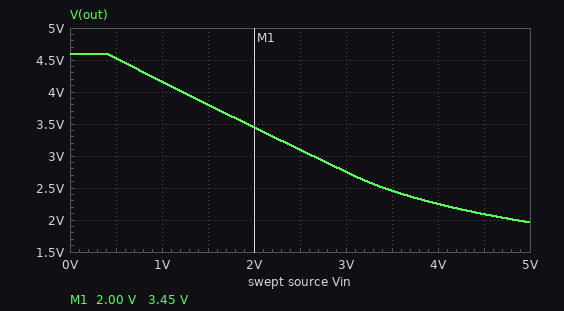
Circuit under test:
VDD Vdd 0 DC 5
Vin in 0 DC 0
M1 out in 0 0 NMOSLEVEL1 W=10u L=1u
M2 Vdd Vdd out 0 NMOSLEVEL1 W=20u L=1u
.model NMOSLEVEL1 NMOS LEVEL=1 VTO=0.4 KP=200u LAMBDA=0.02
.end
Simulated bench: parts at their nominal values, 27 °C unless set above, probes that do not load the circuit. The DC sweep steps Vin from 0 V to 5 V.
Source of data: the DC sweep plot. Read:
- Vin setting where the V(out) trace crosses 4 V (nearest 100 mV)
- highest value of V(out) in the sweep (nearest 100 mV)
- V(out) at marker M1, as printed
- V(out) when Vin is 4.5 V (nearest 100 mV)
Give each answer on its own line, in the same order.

1.2 V
4.6 V
3.45 V
2.1 V
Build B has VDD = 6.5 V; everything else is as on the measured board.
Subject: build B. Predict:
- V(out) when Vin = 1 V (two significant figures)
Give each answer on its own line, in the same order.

5.7 V
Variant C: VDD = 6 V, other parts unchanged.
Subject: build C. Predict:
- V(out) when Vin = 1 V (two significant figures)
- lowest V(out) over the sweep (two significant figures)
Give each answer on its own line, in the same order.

5.2 V
2.7 V
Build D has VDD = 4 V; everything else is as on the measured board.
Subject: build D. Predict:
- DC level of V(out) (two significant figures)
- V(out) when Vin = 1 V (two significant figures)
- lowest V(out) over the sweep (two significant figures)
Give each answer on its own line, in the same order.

3.6 V
3.2 V
1.3 V
